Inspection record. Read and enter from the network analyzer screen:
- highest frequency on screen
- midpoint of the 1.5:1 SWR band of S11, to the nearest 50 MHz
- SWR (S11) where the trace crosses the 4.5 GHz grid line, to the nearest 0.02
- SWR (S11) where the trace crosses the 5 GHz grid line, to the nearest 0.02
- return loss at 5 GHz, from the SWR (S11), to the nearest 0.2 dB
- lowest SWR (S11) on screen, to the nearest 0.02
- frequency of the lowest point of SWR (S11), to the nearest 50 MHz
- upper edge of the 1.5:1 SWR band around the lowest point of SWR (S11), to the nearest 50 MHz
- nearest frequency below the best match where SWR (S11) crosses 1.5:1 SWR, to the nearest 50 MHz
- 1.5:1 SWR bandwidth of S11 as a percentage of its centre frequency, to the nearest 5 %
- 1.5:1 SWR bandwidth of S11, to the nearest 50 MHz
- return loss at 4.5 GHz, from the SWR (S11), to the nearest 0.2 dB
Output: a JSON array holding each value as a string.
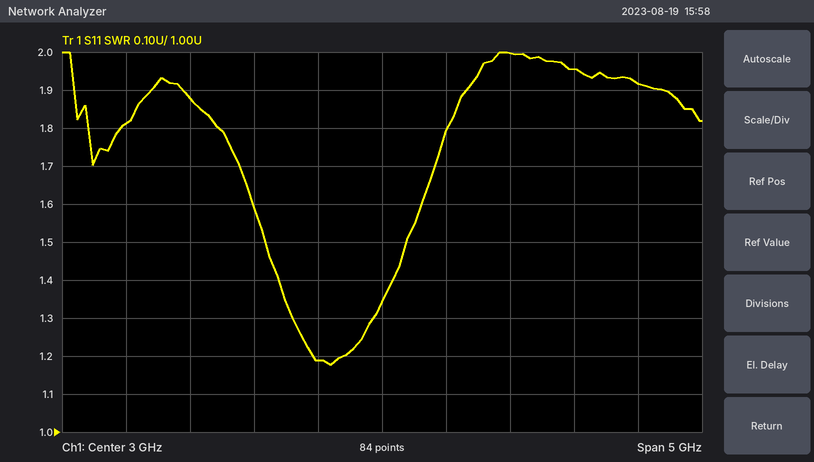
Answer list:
["5.5 GHz", "2.65 GHz", "1.96", "1.92", "10.0 dB", "1.18", "2.60 GHz", "3.20 GHz", "2.10 GHz", "40 %", "1.10 GHz", "9.8 dB"]
